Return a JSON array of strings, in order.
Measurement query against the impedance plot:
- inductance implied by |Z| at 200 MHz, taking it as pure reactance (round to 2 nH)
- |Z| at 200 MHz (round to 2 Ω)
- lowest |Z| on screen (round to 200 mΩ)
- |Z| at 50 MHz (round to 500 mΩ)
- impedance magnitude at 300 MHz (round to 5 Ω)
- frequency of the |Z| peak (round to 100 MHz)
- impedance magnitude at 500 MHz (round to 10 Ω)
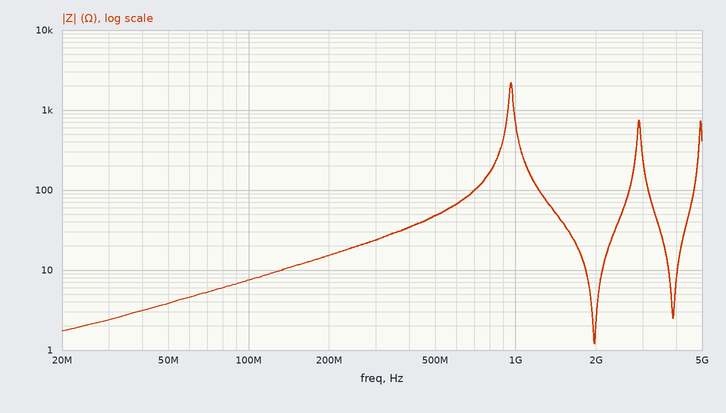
["12 nH", "16 Ω", "1.2 Ω", "4.0 Ω", "25 Ω", "1.0 GHz", "50 Ω"]
